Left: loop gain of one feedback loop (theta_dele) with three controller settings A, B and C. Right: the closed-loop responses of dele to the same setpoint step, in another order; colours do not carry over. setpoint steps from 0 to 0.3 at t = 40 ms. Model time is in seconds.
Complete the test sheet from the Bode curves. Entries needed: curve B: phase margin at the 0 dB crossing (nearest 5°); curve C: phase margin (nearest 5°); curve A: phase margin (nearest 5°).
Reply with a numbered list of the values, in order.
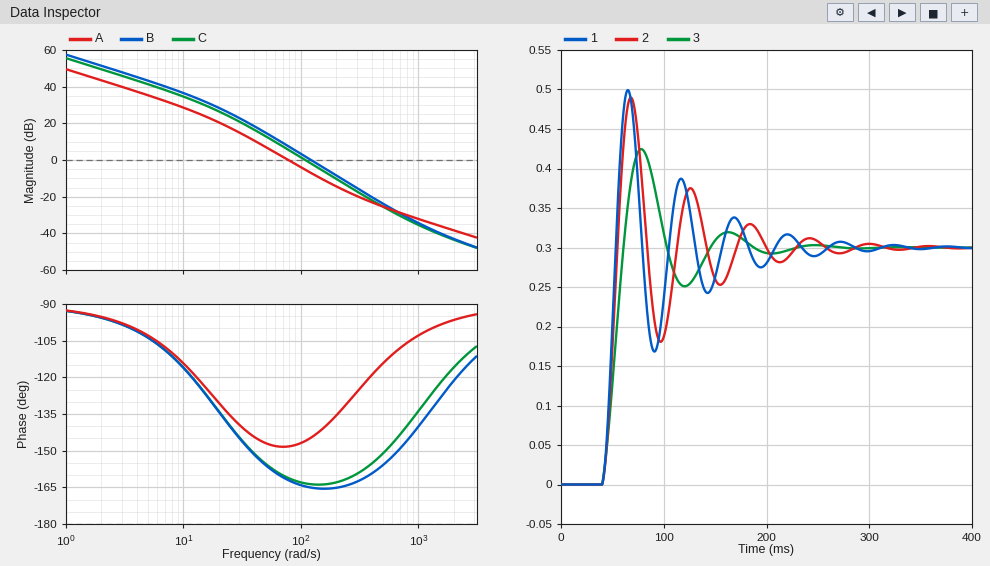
1. 15°
2. 15°
3. 30°
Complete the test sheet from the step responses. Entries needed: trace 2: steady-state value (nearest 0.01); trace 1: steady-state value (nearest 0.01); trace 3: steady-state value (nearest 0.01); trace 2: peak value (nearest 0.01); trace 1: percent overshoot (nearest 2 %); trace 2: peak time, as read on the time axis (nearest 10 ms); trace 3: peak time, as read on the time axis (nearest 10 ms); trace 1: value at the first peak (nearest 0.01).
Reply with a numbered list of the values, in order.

1. 0.30
2. 0.30
3. 0.30
4. 0.49
5. 66 %
6. 70 ms
7. 80 ms
8. 0.50
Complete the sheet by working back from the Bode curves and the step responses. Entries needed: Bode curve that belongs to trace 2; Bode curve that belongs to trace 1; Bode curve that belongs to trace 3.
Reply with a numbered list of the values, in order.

1. C
2. B
3. A
